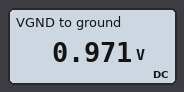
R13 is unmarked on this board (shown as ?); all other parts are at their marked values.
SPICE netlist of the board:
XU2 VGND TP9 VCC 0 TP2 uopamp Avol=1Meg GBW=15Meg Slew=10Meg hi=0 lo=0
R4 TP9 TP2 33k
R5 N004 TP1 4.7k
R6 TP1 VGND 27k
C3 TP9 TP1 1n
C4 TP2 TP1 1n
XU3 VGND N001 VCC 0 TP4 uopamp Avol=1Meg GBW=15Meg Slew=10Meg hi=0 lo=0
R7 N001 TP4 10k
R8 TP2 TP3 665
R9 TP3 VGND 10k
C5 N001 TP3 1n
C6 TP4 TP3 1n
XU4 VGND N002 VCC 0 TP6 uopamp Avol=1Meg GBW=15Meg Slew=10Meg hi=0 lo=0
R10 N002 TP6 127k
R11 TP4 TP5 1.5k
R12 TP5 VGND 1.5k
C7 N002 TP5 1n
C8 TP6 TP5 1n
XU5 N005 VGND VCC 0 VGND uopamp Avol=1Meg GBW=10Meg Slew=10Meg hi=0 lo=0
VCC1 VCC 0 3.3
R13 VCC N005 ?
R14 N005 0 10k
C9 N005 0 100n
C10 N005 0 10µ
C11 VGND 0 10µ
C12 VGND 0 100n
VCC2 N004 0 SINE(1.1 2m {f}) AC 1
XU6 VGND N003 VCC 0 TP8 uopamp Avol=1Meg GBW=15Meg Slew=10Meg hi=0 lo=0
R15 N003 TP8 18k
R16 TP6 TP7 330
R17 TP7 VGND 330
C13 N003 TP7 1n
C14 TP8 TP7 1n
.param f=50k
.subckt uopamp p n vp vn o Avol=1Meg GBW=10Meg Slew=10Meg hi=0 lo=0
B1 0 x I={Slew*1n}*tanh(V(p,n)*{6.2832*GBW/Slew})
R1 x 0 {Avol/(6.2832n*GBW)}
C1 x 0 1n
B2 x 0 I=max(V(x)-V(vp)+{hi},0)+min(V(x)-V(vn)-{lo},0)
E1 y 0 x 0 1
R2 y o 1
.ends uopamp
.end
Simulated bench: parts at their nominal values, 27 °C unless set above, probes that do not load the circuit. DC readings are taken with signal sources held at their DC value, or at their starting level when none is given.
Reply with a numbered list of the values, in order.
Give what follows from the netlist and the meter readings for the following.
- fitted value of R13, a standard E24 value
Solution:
1. 24 kΩ
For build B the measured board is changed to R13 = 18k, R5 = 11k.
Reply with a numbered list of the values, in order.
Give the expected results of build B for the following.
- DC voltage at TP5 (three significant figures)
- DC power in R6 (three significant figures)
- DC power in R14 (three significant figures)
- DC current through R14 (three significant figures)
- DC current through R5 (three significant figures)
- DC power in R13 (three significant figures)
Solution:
1. 1.18 V
2. 115 nW
3. 139 µW
4. 118 µA
5. 2.07 µA
6. 250 µW
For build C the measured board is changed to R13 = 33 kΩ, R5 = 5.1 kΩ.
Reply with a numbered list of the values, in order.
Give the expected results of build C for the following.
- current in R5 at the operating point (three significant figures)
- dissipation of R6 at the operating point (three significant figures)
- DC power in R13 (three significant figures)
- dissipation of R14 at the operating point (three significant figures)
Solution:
1. 10.4 µA
2. 2.90 µW
3. 194 µW
4. 58.9 µW
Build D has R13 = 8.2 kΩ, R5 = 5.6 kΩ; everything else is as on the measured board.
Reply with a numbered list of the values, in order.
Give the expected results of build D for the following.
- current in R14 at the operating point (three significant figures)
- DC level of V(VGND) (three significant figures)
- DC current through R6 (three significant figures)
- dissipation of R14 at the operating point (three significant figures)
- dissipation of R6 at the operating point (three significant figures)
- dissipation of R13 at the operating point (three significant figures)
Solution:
1. 181 µA
2. 1.81 V
3. 21.9 µA
4. 329 µW
5. 12.9 µW
6. 270 µW
